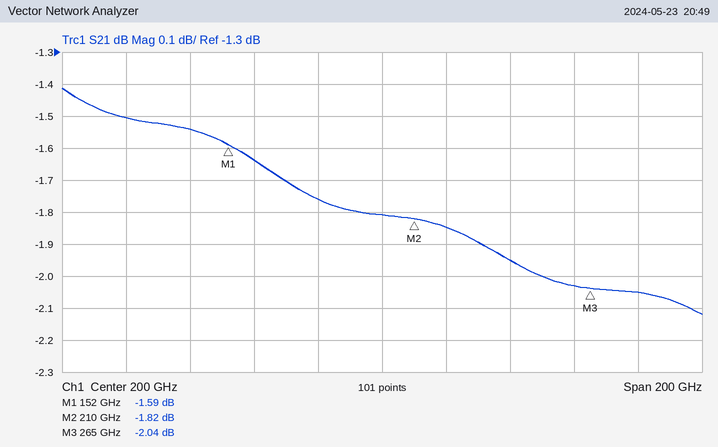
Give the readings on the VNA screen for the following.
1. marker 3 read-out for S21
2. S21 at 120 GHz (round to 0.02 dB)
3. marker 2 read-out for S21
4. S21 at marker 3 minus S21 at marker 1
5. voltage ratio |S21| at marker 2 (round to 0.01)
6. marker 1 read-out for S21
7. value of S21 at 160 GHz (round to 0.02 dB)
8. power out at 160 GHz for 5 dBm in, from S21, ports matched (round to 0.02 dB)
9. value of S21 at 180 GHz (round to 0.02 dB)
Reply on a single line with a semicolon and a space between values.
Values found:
-2.04 dB; -1.50 dB; -1.82 dB; -0.45 dB; 0.81; -1.59 dB; -1.64 dB; 3.36 dBm; -1.76 dB
